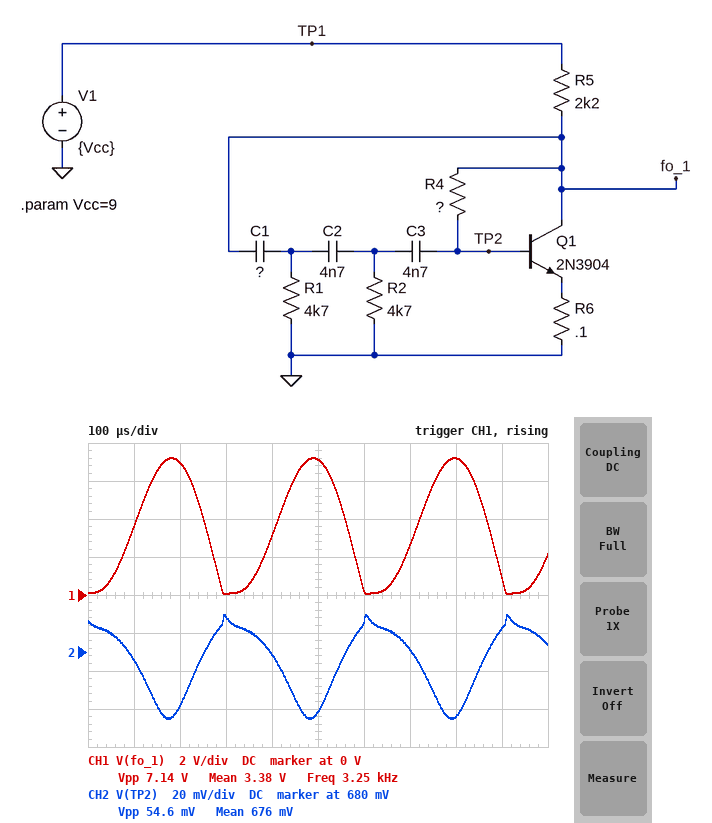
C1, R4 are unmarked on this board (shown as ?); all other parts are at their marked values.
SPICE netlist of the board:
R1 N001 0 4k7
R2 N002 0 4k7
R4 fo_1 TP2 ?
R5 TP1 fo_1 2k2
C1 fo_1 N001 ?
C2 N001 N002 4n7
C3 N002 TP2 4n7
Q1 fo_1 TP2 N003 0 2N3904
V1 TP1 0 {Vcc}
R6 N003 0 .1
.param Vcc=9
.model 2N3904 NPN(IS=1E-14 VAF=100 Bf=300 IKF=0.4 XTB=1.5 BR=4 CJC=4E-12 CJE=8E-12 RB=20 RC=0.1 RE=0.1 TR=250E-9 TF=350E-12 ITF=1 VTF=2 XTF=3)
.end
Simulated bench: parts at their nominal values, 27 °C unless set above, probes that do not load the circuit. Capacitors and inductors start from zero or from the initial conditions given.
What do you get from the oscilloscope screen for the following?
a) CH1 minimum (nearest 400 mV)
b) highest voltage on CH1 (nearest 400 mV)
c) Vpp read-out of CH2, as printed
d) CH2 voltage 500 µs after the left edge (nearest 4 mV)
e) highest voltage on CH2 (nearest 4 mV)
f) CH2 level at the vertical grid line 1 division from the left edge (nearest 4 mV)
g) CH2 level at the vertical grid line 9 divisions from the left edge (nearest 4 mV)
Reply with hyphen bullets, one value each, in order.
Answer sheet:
- 0 V
- 7.2 V
- 54.6 mV
- 648 mV
- 700 mV
- 676 mV
- 692 mV
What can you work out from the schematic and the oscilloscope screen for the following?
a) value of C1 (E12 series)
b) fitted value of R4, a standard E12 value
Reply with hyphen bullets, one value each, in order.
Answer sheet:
- 3.9 nF
- 220 kΩ
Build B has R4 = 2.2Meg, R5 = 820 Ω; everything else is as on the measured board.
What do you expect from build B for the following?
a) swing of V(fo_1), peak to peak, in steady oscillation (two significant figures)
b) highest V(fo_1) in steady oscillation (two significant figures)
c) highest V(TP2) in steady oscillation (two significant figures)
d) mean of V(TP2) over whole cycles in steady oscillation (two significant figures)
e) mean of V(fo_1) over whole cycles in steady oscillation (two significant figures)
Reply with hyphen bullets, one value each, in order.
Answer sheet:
- 800 mV
- 8.5 V
- 670 mV
- 650 mV
- 8.1 V
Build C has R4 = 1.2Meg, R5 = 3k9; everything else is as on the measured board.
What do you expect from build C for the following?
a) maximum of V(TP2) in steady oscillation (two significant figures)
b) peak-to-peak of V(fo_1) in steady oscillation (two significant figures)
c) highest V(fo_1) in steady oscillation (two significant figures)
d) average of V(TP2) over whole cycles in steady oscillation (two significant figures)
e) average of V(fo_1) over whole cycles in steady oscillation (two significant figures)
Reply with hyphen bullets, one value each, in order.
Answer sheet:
- 680 mV
- 8.8 V
- 8.9 V
- 600 mV
- 5.2 V
